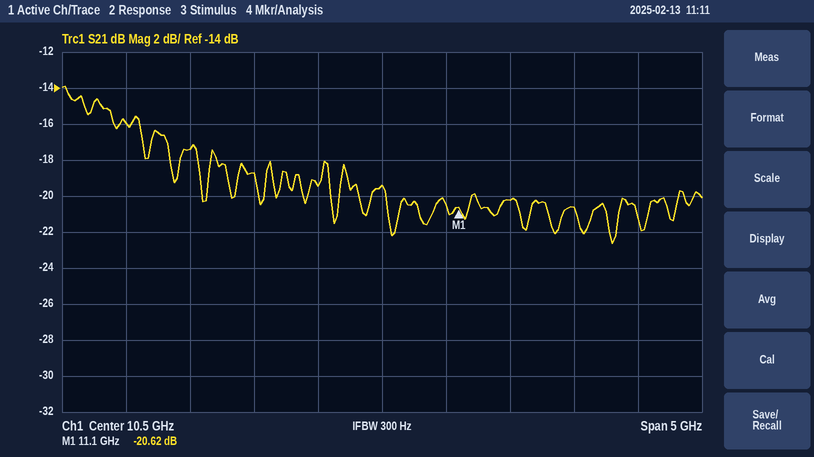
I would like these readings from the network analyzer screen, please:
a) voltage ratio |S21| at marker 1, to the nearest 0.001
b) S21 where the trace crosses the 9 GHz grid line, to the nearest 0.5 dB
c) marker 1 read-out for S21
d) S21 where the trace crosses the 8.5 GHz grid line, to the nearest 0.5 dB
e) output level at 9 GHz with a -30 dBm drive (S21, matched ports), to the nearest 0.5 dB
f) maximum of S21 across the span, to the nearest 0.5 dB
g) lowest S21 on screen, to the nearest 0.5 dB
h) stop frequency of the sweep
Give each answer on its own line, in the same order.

0.093
-17.5 dB
-20.62 dB
-16.0 dB
-47.5 dBm
-14.0 dB
-22.5 dB
13 GHz
